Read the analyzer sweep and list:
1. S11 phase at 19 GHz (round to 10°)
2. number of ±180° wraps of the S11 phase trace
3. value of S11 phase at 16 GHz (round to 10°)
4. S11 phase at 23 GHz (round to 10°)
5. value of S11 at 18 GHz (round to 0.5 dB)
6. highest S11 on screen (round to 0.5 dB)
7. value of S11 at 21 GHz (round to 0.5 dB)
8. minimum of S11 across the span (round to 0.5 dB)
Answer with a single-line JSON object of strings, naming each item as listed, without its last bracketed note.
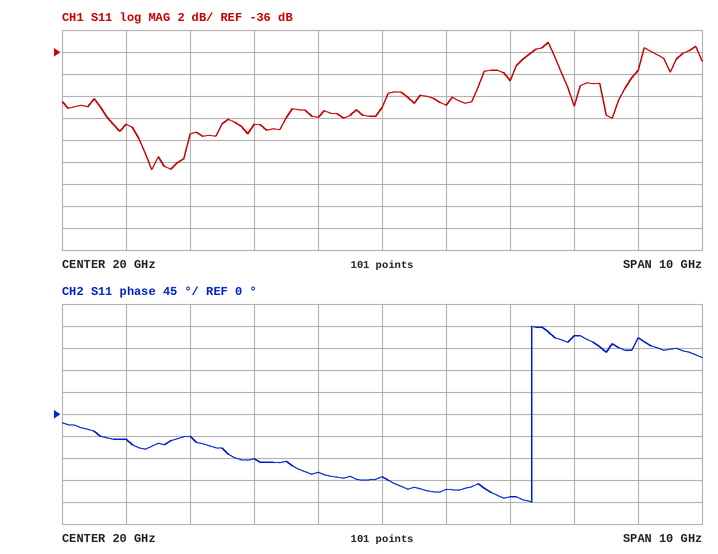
{"S11 phase at 19 GHz": "-120°", "number of ±180° wraps of the S11 phase trace": "1", "value of S11 phase at 16 GHz": "-50°", "S11 phase at 23 GHz": "160°", "value of S11 at 18 GHz": "-42.5 dB", "highest S11 on screen": "-35.0 dB", "value of S11 at 21 GHz": "-41.0 dB", "minimum of S11 across the span": "-46.5 dB"}
